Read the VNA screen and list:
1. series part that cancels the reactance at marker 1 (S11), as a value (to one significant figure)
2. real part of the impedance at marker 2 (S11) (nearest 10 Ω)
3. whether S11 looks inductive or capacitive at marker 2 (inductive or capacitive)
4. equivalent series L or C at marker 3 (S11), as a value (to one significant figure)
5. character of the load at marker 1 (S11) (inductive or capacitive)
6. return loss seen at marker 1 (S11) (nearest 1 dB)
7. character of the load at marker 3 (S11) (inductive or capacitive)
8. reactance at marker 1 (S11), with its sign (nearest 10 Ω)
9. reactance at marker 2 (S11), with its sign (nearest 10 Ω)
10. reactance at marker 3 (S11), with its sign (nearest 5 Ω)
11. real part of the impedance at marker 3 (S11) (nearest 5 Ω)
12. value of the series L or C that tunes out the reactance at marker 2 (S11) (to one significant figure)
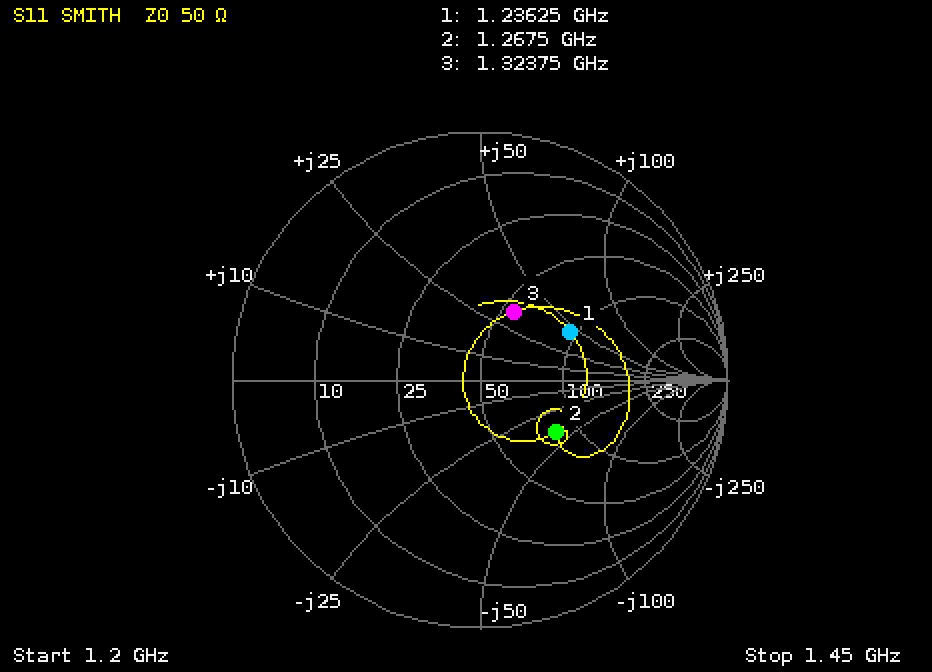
3 pF
80 Ω
capacitive
4 nH
inductive
8 dB
inductive
+40 Ω
-40 Ω
+35 Ω
55 Ω
5 nH
